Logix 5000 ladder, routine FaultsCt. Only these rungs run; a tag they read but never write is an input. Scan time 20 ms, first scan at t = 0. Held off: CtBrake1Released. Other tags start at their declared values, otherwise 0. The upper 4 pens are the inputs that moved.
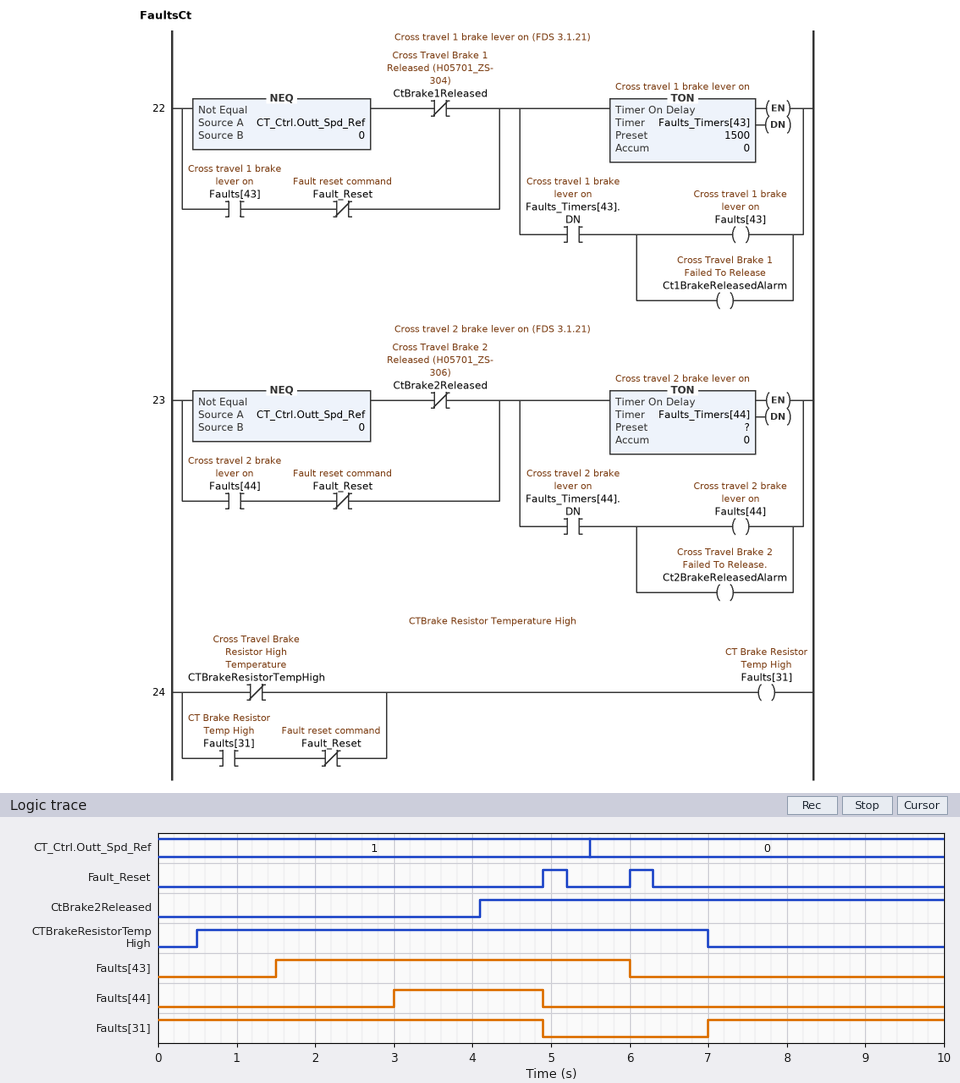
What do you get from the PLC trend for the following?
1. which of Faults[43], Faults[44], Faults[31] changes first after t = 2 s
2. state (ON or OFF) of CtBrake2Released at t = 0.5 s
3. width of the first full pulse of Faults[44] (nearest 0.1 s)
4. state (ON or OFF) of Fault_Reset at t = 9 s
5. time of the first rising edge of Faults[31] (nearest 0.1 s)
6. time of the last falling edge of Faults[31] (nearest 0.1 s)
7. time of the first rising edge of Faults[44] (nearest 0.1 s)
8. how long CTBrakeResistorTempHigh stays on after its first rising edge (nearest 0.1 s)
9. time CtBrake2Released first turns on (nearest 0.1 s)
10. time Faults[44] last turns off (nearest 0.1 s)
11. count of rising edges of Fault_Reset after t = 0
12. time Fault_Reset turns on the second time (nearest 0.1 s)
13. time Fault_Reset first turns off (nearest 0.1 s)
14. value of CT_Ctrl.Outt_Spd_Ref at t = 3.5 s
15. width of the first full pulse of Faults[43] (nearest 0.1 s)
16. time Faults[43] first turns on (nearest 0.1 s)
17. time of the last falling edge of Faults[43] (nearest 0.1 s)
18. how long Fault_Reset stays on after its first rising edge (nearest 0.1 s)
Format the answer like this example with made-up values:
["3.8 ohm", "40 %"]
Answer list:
["Faults[44]", "OFF", "1.9 s", "OFF", "7.0 s", "4.9 s", "3.0 s", "6.5 s", "4.1 s", "4.9 s", "2", "6.0 s", "5.2 s", "1", "4.5 s", "1.5 s", "6.0 s", "0.3 s"]
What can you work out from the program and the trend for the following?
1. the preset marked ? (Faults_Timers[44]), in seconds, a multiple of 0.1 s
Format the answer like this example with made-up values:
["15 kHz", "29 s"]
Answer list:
["3.0 s"]
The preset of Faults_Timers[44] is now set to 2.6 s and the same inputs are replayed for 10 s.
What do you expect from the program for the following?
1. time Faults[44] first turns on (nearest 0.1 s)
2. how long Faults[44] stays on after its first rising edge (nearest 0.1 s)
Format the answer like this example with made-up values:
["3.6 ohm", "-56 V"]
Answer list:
["2.6 s", "2.3 s"]
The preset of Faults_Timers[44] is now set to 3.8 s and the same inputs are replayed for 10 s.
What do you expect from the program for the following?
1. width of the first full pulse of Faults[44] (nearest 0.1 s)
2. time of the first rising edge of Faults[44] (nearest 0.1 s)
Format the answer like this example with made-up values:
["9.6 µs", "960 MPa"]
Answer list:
["1.1 s", "3.8 s"]
